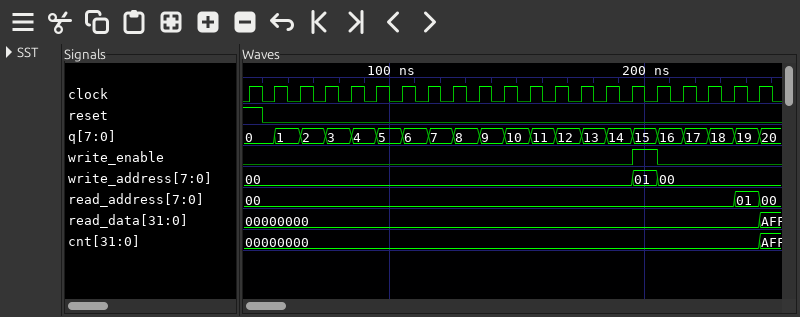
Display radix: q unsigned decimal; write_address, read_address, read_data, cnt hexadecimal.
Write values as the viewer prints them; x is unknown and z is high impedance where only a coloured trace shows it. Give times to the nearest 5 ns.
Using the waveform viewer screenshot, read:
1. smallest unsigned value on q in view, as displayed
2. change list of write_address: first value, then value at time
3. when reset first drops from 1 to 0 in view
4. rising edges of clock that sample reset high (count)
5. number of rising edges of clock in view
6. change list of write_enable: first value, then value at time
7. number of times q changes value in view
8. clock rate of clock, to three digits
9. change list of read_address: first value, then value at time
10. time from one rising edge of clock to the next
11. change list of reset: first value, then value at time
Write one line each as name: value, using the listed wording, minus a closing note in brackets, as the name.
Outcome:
smallest unsigned value on q in view, as displayed: 0
change list of write_address: first value, then value at time: 00, 01 at 195 ns, 00 at 205 ns
when reset first drops from 1 to 0 in view: 50 ns
rising edges of clock that sample reset high: 1
number of rising edges of clock in view: 21
change list of write_enable: first value, then value at time: 0, 1 at 195 ns, 0 at 205 ns
number of times q changes value in view: 20
clock rate of clock, to three digits: 100 MHz
change list of read_address: first value, then value at time: 00, 01 at 235 ns, 00 at 245 ns
time from one rising edge of clock to the next: 10 ns
change list of reset: first value, then value at time: 1, 0 at 50 ns
